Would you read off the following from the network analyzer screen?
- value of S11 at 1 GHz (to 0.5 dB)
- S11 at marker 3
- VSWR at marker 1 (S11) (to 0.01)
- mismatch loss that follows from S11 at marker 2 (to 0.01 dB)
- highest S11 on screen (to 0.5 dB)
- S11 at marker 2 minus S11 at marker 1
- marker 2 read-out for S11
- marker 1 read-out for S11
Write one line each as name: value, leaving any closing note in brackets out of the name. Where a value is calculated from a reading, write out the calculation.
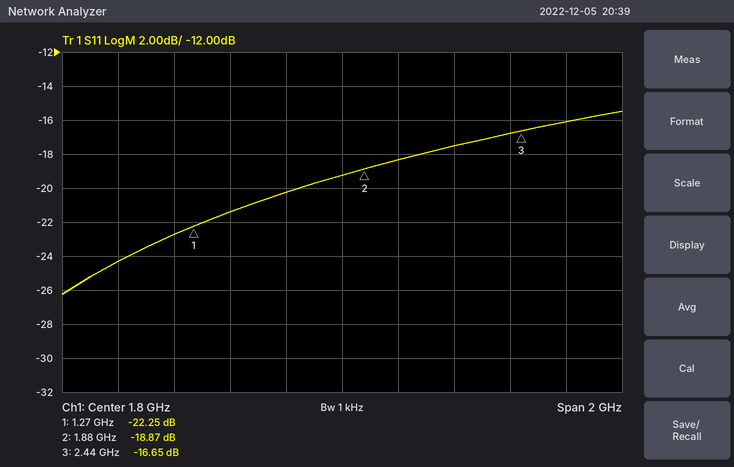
value of S11 at 1 GHz: -24.5 dB
S11 at marker 3: -16.65 dB
VSWR at marker 1 (S11): (1 + 0.0772)/(1 − 0.0772) ≈ 1.17
mismatch loss that follows from S11 at marker 2: −10 log10(1 − 10^(-18.87/10)) ≈ 0.06 dB
highest S11 on screen: -15.5 dB
S11 at marker 2 minus S11 at marker 1: -18.87 − (-22.25) = 3.38 dB
marker 2 read-out for S11: -18.87 dB
marker 1 read-out for S11: -22.25 dB
